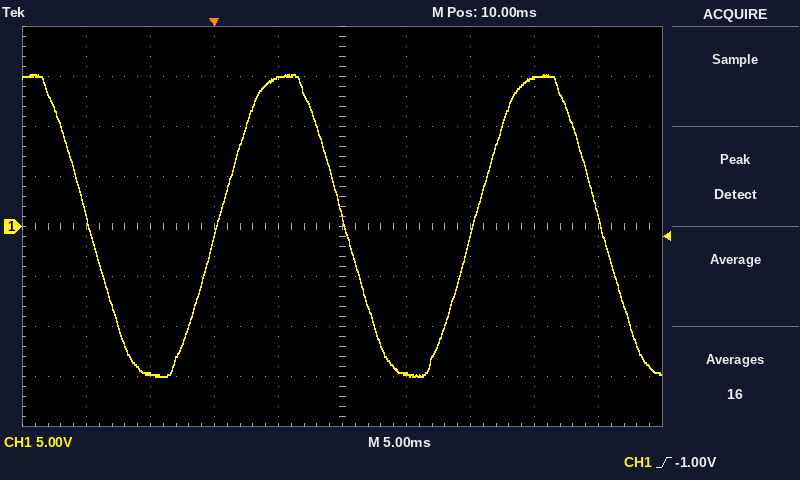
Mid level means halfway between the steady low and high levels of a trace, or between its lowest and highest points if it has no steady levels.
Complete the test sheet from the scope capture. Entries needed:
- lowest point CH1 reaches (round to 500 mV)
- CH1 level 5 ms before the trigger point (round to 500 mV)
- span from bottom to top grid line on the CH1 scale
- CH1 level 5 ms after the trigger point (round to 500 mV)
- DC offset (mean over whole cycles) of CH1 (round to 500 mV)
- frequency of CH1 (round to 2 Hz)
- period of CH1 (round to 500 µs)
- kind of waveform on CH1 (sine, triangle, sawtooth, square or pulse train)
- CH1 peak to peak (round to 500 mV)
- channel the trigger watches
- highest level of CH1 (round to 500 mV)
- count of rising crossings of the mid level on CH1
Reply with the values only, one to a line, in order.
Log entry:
-15.0 V
-14.5 V
40 V
15.0 V
0.0 V
50 Hz
20.0 ms
sine
30.0 V
CH1
15.0 V
2
